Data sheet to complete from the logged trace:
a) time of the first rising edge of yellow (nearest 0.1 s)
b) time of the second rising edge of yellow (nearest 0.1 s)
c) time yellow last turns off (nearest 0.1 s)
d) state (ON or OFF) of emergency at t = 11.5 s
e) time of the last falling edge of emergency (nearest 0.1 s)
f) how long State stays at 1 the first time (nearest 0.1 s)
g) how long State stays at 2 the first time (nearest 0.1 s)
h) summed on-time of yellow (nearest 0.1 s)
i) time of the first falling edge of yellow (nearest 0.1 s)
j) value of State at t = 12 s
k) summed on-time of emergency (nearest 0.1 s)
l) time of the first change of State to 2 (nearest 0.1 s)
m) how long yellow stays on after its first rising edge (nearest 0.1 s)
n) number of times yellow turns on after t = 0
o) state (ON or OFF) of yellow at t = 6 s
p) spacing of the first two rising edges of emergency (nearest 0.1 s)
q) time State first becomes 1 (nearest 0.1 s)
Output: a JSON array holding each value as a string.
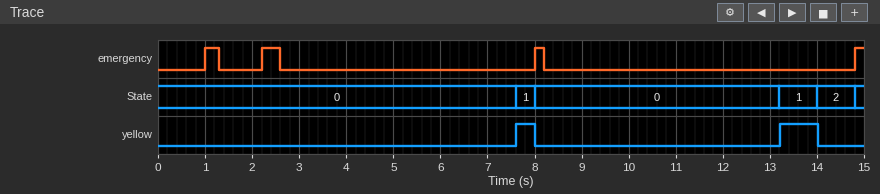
["7.6 s", "13.2 s", "14.0 s", "OFF", "8.2 s", "0.4 s", "0.8 s", "1.2 s", "8.0 s", "0", "1.1 s", "14.0 s", "0.4 s", "2", "OFF", "1.2 s", "7.6 s"]
